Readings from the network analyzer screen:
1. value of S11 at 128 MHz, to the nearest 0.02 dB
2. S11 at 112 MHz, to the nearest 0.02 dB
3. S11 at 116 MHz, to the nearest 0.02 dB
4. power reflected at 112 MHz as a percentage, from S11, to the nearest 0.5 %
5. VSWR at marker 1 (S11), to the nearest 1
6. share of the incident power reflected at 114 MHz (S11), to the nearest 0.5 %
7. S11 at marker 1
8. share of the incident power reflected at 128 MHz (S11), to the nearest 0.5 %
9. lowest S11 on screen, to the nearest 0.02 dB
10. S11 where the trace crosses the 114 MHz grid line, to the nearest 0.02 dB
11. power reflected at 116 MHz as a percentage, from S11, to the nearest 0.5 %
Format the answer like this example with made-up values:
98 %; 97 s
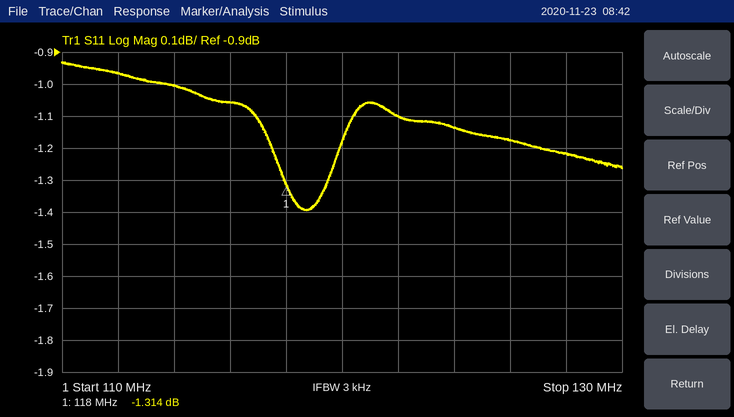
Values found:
-1.22 dB; -0.96 dB; -1.06 dB; 80.0 %; 13; 79.5 %; -1.314 dB; 75.5 %; -1.40 dB; -1.00 dB; 78.5 %
